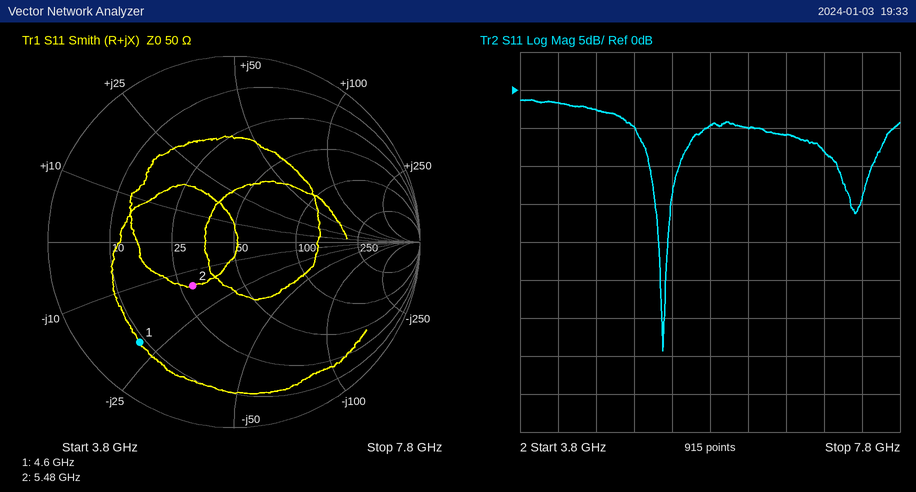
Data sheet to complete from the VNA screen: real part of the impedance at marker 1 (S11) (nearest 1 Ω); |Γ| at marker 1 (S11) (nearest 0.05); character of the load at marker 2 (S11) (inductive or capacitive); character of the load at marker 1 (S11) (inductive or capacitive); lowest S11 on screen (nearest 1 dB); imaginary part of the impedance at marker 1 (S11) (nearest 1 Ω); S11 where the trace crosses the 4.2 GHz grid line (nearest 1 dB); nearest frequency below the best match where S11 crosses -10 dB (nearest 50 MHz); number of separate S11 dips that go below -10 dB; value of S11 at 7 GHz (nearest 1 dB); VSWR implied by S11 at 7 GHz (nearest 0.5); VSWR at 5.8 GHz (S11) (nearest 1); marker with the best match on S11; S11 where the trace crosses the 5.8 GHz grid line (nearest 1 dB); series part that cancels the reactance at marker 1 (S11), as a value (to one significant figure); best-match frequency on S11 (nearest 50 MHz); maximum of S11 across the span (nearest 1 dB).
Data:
9 Ω
0.75
capacitive
capacitive
-34 dB
-21 Ω
-2 dB
5.15 GHz
2
-8 dB
2.5
4
marker 2
-5 dB
700 pH
5.30 GHz
-1 dB
